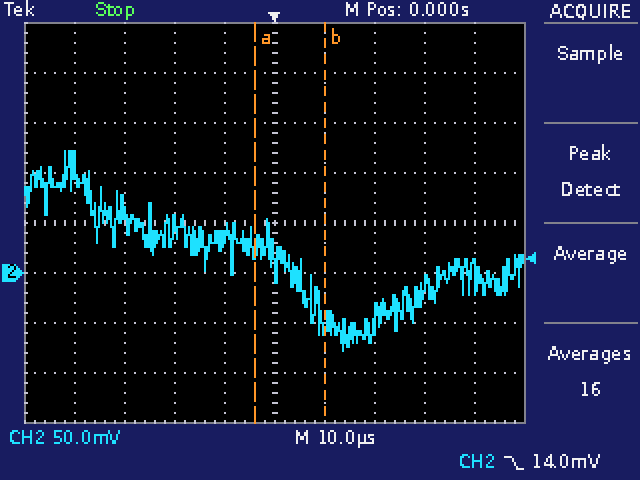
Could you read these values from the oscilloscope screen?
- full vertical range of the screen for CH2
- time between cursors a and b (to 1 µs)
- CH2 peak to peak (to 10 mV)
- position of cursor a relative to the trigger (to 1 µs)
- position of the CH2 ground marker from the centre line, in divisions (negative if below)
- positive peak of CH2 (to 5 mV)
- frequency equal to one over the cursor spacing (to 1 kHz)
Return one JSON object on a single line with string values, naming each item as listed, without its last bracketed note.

{"full vertical range of the screen for CH2": "400 mV", "time between cursors a and b": "14 µs", "CH2 peak to peak": "200 mV", "position of cursor a relative to the trigger": "-4 µs", "position of the CH2 ground marker from the centre line, in divisions": "-1.0 div", "positive peak of CH2": "120 mV", "frequency equal to one over the cursor spacing": "71 kHz"}
